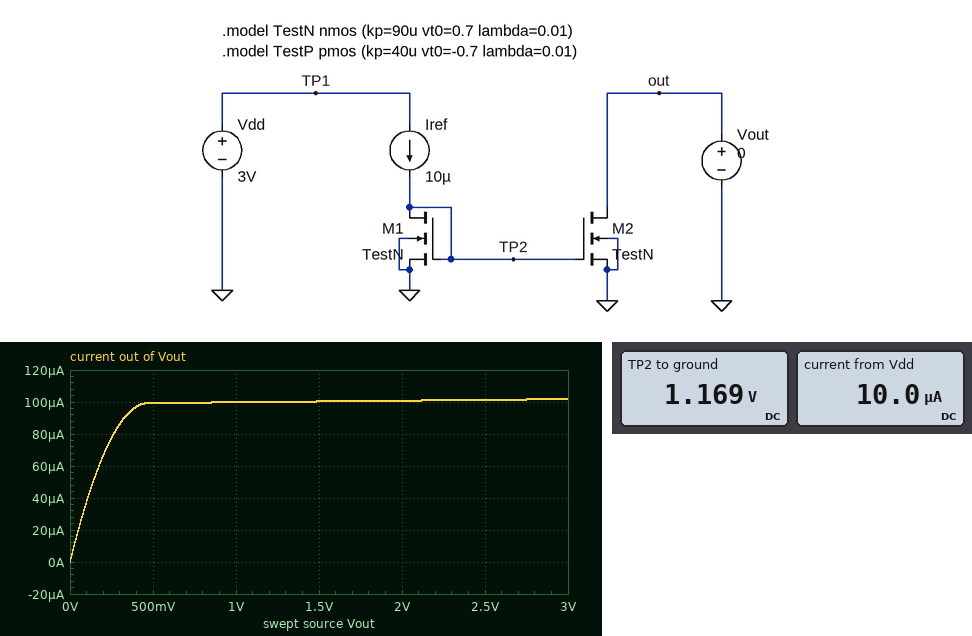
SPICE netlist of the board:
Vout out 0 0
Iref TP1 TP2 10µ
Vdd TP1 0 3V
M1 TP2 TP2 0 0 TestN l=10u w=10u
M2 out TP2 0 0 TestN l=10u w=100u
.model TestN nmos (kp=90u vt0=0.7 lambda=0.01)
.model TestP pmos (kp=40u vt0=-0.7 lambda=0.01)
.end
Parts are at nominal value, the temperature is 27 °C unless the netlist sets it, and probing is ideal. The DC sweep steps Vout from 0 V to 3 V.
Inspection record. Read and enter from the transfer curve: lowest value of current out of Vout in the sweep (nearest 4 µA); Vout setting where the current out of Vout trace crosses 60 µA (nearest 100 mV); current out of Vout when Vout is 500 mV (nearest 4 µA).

0 A
200 mV
100 µA
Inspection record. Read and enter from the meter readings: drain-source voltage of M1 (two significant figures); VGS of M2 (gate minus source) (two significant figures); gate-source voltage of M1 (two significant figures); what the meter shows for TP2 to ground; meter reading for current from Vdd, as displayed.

1.2 V
1.2 V
1.2 V
1.169 V
10.0 µA
